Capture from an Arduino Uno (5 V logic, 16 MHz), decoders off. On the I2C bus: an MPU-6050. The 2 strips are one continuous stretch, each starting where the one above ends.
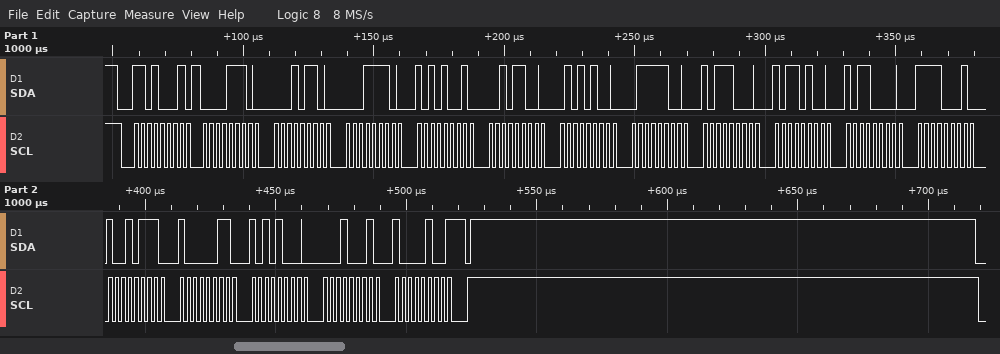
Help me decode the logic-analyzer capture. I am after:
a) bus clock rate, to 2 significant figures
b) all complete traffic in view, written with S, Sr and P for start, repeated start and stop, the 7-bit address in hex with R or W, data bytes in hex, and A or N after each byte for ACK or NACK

400 kHz
S 68R A 0E A 16 A 1E A A9 A 2C A 54 A 7C A B8 A B4 A B0 A F1 A 97 A 83 A A8 A 11 A 84 N P
